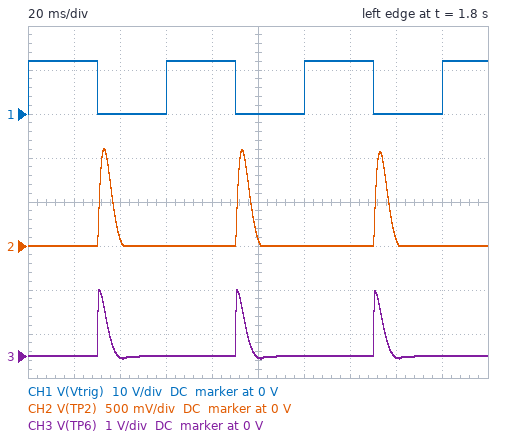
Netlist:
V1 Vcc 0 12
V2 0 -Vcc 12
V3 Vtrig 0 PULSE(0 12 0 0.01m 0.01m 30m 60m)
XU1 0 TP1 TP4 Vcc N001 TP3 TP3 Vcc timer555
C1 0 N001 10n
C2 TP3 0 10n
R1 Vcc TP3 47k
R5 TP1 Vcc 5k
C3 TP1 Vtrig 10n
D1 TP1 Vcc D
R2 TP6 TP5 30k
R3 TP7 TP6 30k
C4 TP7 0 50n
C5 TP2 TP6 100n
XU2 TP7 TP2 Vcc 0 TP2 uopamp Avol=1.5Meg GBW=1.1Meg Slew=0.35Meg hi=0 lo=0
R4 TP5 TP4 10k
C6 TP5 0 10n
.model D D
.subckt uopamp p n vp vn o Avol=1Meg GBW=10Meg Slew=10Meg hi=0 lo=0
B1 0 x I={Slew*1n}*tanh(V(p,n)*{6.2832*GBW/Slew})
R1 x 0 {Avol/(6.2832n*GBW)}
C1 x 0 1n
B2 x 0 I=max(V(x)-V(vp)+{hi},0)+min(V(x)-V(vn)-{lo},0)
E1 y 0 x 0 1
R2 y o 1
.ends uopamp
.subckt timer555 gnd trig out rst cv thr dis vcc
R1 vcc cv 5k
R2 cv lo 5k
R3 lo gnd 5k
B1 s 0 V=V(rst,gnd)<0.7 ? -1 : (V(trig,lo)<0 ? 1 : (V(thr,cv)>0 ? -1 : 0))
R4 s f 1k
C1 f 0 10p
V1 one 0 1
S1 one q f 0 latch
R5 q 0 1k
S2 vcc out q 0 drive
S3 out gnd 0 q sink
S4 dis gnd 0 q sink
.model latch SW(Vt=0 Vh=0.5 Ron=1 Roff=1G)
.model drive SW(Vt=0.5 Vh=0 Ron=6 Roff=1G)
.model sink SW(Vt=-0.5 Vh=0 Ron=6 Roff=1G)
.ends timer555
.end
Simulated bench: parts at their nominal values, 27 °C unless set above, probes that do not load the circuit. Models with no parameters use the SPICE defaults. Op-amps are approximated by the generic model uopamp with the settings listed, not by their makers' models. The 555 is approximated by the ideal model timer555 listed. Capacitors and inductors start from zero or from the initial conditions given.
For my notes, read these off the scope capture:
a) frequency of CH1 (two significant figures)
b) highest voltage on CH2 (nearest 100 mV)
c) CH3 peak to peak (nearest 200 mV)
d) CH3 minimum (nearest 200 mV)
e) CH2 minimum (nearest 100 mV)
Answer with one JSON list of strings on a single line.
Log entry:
["17 Hz", "1.1 V", "1.6 V", "0 V", "0 V"]
